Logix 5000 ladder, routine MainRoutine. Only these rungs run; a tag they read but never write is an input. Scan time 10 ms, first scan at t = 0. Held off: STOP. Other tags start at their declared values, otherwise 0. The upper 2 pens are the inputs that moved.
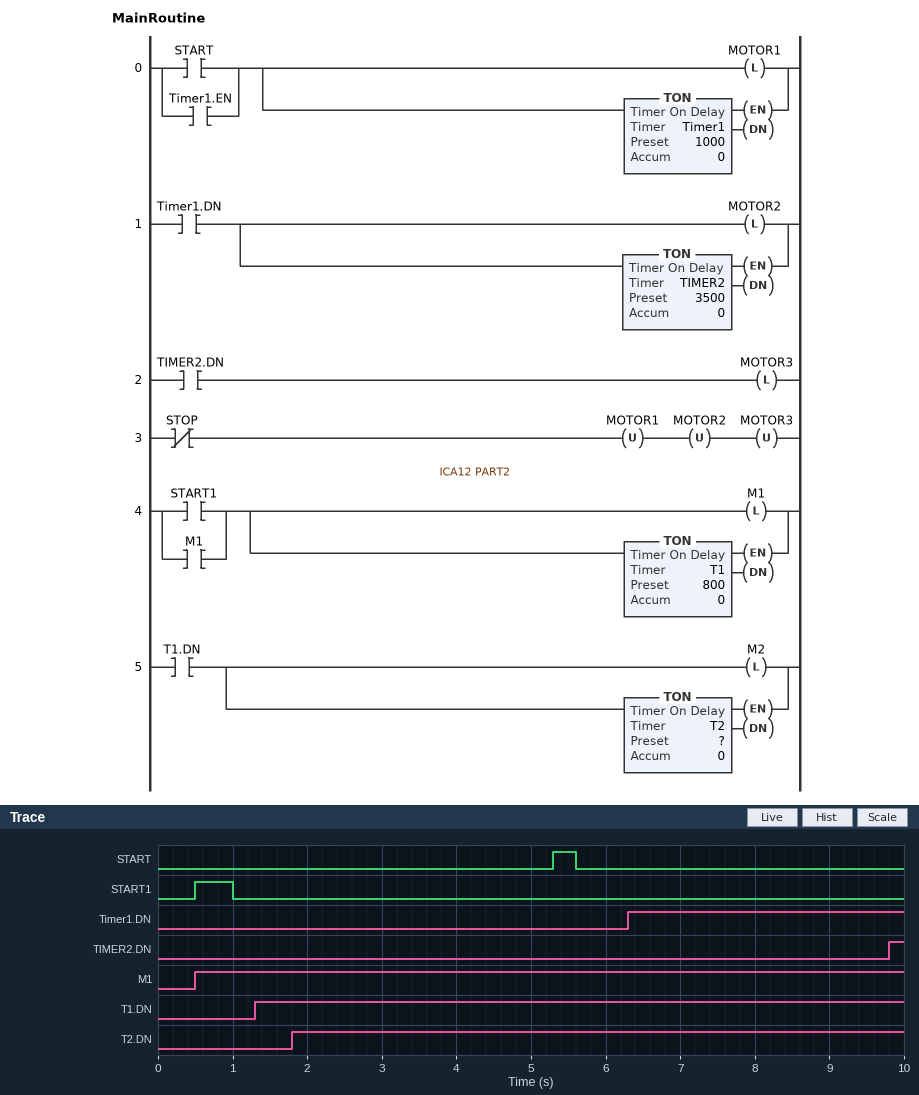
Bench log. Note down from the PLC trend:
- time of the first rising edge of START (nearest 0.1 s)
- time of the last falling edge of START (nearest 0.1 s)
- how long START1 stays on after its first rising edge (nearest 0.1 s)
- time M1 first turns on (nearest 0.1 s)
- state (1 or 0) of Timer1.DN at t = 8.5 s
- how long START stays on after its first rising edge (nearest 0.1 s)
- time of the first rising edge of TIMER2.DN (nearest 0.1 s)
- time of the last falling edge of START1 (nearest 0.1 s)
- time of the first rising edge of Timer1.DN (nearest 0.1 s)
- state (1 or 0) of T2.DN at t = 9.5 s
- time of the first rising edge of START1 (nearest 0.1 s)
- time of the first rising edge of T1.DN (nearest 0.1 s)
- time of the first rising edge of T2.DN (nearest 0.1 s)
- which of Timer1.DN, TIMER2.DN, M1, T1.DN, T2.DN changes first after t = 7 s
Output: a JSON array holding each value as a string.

["5.3 s", "5.6 s", "0.5 s", "0.5 s", "1", "0.3 s", "9.8 s", "1.0 s", "6.3 s", "1", "0.5 s", "1.3 s", "1.8 s", "TIMER2.DN"]
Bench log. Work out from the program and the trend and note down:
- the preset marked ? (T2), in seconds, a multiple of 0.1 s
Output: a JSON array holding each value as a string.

["0.5 s"]
